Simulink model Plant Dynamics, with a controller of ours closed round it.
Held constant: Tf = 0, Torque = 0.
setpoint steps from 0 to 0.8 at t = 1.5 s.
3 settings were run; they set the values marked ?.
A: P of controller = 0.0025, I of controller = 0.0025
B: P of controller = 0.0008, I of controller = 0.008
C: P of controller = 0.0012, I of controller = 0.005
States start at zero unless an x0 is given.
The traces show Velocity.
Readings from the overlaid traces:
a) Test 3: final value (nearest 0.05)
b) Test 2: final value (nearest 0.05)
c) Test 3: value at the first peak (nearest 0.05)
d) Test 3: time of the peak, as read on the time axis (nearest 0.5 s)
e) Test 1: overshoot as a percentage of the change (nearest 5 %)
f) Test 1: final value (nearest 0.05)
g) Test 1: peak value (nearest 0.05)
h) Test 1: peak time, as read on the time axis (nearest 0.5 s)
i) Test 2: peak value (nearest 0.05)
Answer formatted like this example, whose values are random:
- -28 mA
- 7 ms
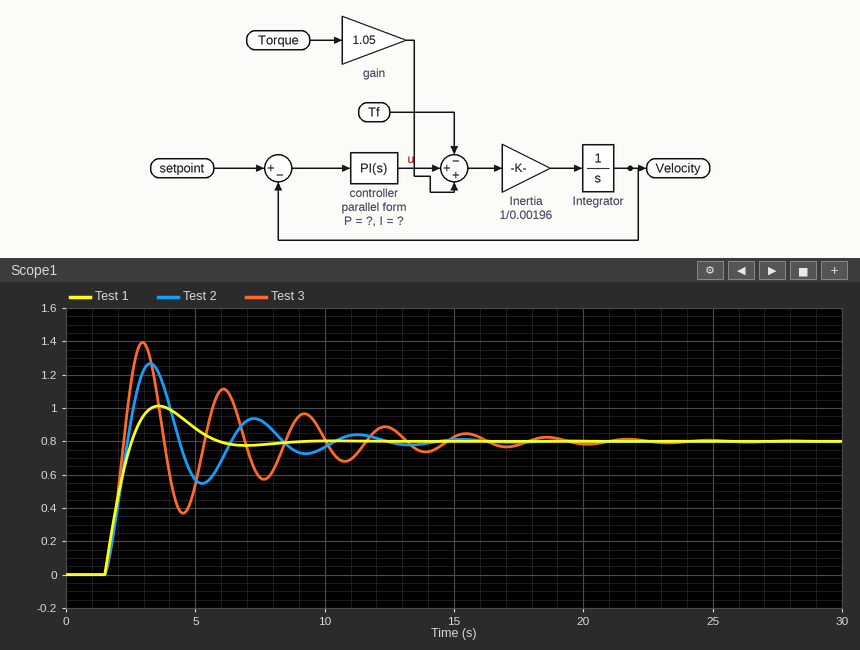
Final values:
- 0.80
- 0.80
- 1.40
- 3.0 s
- 25 %
- 0.80
- 1.00
- 3.5 s
- 1.25
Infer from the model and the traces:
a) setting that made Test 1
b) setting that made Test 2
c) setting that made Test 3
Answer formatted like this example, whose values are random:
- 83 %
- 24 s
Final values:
- A
- C
- B
